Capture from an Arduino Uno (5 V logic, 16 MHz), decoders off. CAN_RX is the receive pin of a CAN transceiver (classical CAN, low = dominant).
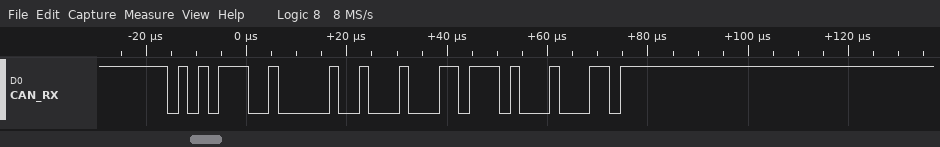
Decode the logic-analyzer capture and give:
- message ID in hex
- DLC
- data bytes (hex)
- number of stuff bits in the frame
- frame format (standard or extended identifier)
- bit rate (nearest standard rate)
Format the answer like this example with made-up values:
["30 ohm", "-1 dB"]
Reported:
["0x572", "1", "11", "1", "standard", "500 kbit/s"]
